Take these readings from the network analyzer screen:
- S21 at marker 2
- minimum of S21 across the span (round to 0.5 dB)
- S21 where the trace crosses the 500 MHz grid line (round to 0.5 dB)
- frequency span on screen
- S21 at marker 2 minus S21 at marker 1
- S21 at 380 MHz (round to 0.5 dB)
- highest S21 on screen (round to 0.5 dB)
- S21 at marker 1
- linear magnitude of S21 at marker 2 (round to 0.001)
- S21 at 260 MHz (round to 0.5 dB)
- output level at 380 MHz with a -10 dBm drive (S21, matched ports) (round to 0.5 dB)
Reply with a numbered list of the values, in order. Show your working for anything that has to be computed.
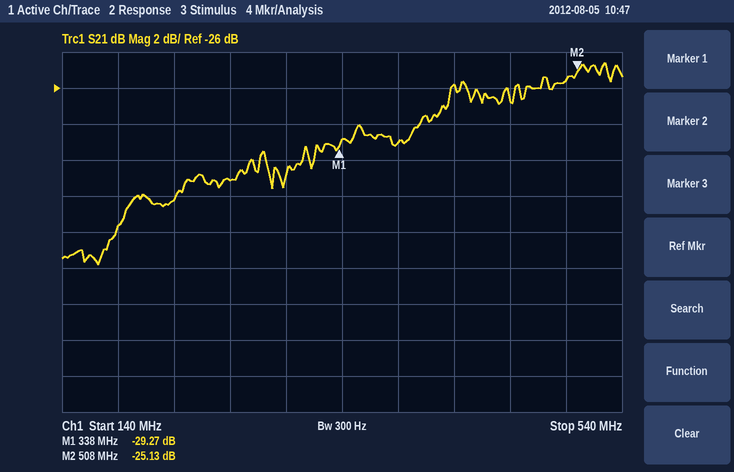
1. -25.13 dB
2. -36.0 dB
3. -25.5 dB
4. 400 MHz
5. -25.13 − (-29.27) = 4.14 dB
6. -29.0 dB
7. -24.5 dB
8. -29.27 dB
9. 10^(-25.13/20) ≈ 0.055
10. -31.0 dB
11. -10 dBm + (-29.0 dB) = -39.0 dBm
